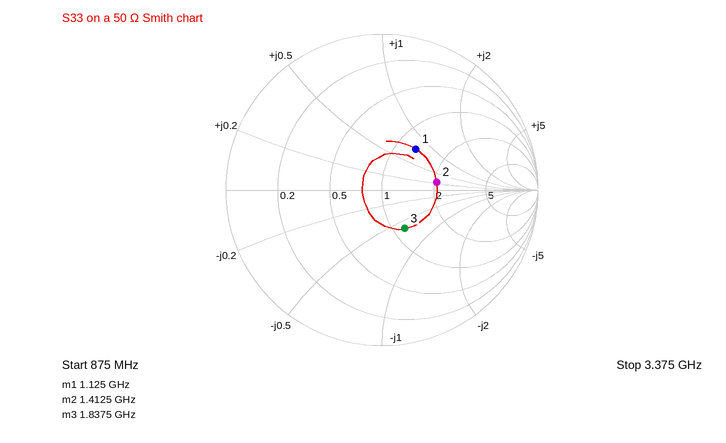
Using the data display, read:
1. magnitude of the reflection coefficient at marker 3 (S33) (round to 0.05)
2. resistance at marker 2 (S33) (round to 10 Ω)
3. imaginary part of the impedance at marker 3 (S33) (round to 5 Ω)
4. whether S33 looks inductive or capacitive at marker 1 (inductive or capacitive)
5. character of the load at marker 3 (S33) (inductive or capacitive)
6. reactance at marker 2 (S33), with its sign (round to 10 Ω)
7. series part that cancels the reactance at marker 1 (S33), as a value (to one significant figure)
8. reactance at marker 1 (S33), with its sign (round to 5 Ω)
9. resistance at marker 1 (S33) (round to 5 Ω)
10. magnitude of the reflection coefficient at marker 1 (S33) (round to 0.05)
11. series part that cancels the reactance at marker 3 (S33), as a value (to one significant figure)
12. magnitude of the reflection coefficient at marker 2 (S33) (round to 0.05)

0.30
100 Ω
-30 Ω
inductive
capacitive
+10 Ω
4 pF
+40 Ω
65 Ω
0.35
3 nH
0.35
